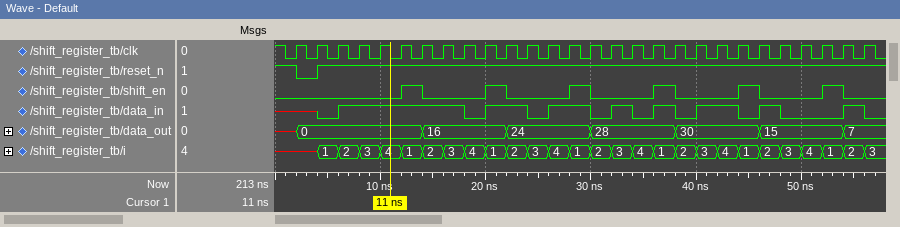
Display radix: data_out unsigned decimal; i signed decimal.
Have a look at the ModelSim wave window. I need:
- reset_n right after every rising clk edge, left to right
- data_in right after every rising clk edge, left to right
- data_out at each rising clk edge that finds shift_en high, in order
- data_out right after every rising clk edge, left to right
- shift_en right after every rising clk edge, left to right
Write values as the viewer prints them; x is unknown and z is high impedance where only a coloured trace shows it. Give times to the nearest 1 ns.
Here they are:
0 1 1 1 1 1 1 1 1 1 1 1 1 1 1 1 1 1 1 1 1 1 1 1 1 1 1 1
x 0 1 1 1 1 1 1 0 1 1 0 1 1 0 1 0 1 0 1 1 0 1 0 0 0 1 0
0, 16, 24, 28, 30, 15
0, 0, 0, 0, 0, 0, 16, 16, 16, 16, 24, 24, 24, 24, 28, 28, 28, 28, 30, 30, 30, 30, 15, 15, 15, 15, 7, 7
0 0 0 0 0 1 0 0 0 1 0 0 0 1 0 0 0 1 0 0 0 1 0 0 0 1 0 0
